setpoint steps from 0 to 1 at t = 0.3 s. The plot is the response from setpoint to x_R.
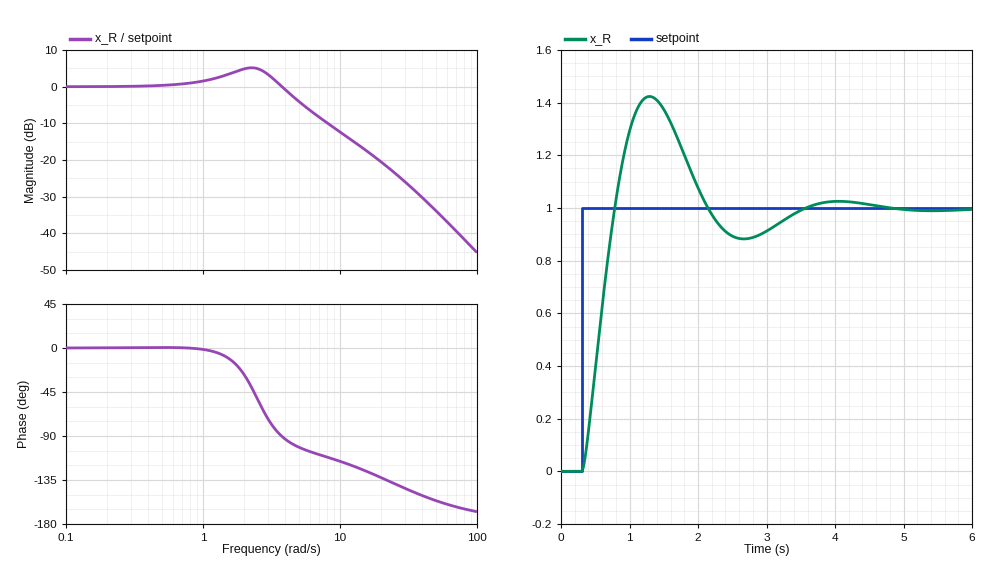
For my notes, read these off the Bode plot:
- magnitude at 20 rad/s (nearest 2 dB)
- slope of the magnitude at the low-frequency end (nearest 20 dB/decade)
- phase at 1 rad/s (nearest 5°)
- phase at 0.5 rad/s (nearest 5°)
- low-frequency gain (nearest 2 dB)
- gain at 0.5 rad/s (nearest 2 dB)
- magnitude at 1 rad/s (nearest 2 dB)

-20 dB
0 dB/decade
0°
0°
0 dB
0 dB
2 dB
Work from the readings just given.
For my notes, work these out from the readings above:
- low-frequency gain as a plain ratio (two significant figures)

1.0
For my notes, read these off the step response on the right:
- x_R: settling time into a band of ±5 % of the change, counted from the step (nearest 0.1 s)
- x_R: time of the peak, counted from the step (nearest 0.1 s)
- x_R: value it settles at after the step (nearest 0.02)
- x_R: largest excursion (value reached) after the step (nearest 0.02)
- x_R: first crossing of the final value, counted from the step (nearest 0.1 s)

2.9 s
1.0 s
1.00
1.42
0.5 s
